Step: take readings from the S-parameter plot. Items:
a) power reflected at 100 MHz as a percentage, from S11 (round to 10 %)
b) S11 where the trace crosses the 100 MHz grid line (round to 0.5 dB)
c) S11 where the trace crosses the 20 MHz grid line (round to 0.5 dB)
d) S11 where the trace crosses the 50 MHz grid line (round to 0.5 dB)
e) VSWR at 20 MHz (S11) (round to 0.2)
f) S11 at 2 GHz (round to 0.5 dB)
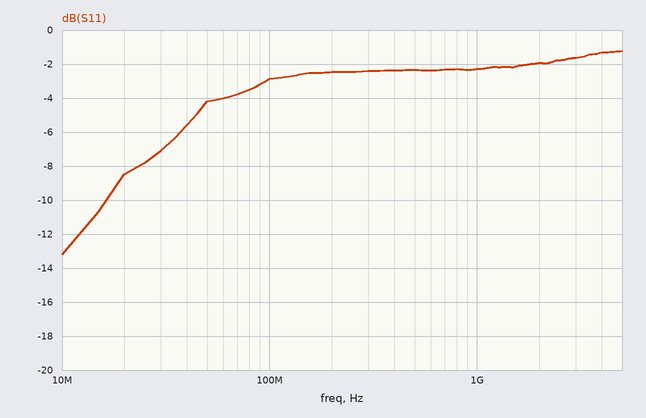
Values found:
50 %
-3.0 dB
-8.5 dB
-4.0 dB
2.2
-2.0 dB
